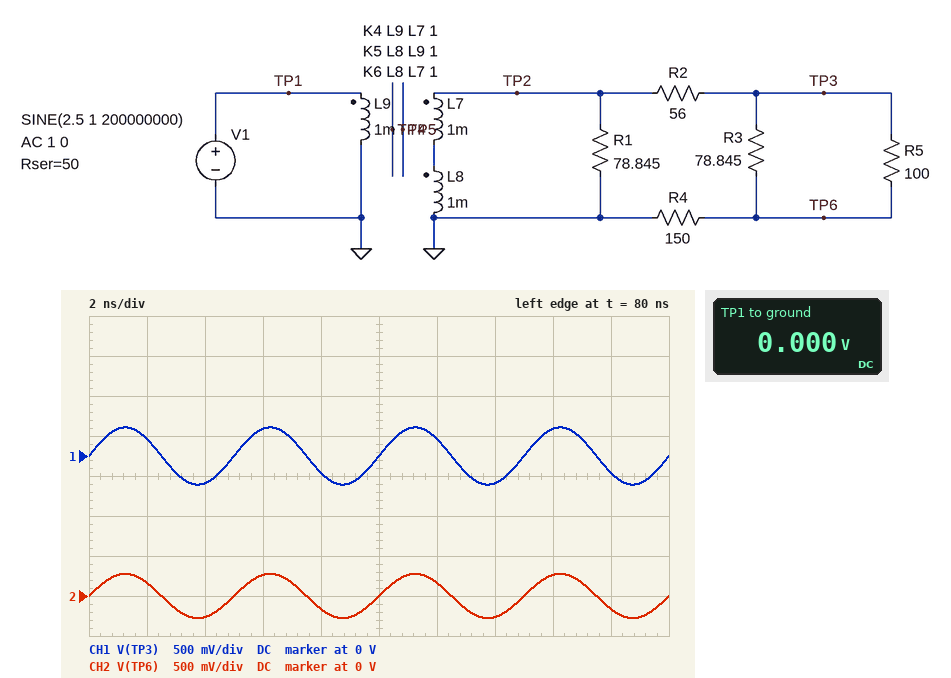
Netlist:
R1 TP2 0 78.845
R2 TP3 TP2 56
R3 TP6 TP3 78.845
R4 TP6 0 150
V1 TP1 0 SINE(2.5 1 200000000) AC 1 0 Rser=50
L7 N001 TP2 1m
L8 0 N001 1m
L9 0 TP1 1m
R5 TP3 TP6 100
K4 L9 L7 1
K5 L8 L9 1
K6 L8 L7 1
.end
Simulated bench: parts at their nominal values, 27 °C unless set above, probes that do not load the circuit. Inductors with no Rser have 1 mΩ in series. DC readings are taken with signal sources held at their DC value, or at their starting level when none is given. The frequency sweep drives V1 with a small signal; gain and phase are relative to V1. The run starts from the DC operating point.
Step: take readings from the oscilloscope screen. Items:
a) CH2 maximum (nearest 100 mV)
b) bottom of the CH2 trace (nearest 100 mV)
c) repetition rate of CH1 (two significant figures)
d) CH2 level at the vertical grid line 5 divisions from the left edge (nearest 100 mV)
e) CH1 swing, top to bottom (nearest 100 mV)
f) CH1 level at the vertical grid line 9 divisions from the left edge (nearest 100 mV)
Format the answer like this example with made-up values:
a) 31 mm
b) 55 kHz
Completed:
a) 300 mV
b) -300 mV
c) 200 MHz
d) 0 V
e) 700 mV
f) -200 mV
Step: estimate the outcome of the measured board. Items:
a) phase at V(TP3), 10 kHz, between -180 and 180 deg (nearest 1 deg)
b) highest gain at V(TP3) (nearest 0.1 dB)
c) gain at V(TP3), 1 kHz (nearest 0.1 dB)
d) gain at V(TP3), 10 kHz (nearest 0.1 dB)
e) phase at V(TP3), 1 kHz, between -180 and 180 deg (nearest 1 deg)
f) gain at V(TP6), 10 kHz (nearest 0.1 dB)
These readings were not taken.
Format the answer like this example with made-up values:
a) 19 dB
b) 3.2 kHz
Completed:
a) 10 deg
b) -8.9 dB
c) -15.3 dB
d) -9.1 dB
e) 61 deg
f) -11.3 dB
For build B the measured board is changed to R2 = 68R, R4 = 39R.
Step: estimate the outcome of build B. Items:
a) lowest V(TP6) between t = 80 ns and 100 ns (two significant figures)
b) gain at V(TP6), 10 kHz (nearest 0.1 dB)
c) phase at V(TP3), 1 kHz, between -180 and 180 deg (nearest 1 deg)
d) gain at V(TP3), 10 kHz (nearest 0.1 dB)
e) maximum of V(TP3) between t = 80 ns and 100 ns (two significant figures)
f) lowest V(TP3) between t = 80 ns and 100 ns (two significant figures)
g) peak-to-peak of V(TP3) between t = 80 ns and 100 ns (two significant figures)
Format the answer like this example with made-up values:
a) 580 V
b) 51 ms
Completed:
a) -110 mV
b) -19.6 dB
c) 59 deg
d) -13.0 dB
e) 230 mV
f) -230 mV
g) 450 mV
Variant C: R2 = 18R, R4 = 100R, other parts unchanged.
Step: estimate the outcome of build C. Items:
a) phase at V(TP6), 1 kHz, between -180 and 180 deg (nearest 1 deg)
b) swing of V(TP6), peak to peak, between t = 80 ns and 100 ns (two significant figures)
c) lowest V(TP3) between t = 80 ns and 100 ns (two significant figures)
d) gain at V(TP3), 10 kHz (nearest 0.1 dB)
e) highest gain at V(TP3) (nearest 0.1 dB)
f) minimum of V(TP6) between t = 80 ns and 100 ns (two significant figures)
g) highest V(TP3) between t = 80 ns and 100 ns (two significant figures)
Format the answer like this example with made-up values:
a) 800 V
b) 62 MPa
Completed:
a) 59 deg
b) 520 mV
c) -370 mV
d) -8.7 dB
e) -8.6 dB
f) -260 mV
g) 370 mV
